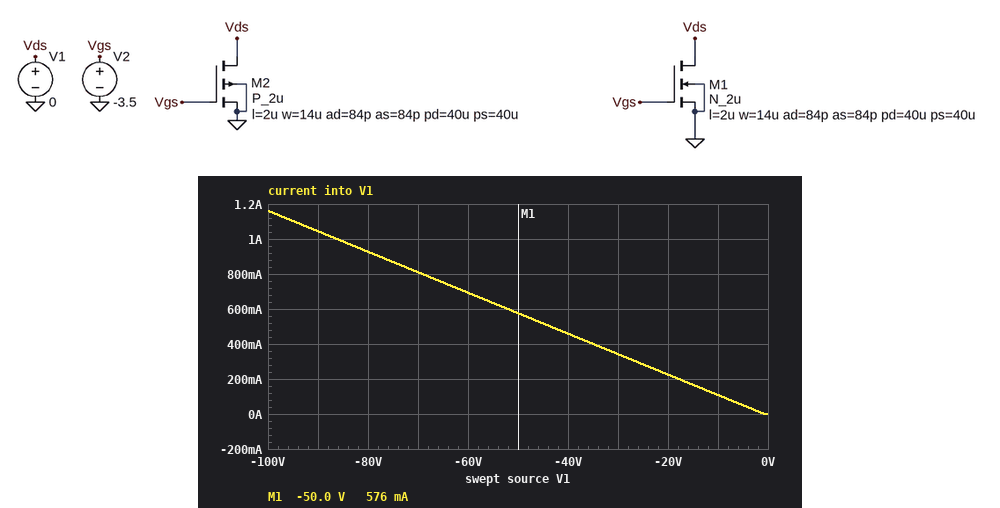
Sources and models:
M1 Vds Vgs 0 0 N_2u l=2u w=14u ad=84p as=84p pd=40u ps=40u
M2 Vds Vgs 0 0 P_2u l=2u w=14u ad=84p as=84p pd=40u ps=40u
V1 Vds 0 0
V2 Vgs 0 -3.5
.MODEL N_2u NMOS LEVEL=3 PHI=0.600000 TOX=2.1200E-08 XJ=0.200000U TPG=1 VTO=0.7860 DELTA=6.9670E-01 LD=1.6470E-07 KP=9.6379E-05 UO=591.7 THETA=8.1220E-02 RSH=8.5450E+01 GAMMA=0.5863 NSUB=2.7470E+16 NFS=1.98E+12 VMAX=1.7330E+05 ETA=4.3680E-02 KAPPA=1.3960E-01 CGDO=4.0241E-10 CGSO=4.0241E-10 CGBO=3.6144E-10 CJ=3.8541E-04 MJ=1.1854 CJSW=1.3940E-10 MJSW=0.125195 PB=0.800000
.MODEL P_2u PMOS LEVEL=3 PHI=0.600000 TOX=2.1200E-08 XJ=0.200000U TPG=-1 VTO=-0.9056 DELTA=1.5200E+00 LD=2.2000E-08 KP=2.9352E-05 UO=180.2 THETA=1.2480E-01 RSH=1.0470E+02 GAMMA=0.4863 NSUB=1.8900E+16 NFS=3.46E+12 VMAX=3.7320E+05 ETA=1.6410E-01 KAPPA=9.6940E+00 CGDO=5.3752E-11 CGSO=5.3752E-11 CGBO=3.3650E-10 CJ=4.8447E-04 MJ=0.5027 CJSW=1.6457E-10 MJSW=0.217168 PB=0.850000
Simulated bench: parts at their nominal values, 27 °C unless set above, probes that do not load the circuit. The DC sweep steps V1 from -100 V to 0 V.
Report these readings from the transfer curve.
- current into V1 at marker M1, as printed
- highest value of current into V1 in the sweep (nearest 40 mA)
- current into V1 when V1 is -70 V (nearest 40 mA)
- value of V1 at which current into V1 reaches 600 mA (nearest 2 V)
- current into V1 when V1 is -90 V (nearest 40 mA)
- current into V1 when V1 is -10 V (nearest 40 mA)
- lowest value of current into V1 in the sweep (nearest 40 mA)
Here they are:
576 mA
1.16 A
800 mA
-52 V
1.04 A
120 mA
0 A
